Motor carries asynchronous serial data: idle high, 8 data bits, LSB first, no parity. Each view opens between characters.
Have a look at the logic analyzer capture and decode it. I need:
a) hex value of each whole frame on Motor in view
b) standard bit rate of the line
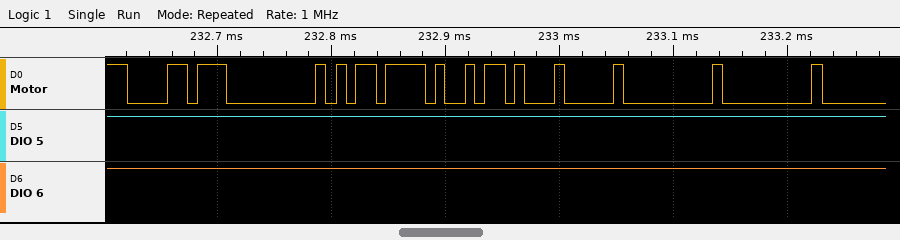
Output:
D8, 00, ED, 69, 04, 00, 00
115200 baud
